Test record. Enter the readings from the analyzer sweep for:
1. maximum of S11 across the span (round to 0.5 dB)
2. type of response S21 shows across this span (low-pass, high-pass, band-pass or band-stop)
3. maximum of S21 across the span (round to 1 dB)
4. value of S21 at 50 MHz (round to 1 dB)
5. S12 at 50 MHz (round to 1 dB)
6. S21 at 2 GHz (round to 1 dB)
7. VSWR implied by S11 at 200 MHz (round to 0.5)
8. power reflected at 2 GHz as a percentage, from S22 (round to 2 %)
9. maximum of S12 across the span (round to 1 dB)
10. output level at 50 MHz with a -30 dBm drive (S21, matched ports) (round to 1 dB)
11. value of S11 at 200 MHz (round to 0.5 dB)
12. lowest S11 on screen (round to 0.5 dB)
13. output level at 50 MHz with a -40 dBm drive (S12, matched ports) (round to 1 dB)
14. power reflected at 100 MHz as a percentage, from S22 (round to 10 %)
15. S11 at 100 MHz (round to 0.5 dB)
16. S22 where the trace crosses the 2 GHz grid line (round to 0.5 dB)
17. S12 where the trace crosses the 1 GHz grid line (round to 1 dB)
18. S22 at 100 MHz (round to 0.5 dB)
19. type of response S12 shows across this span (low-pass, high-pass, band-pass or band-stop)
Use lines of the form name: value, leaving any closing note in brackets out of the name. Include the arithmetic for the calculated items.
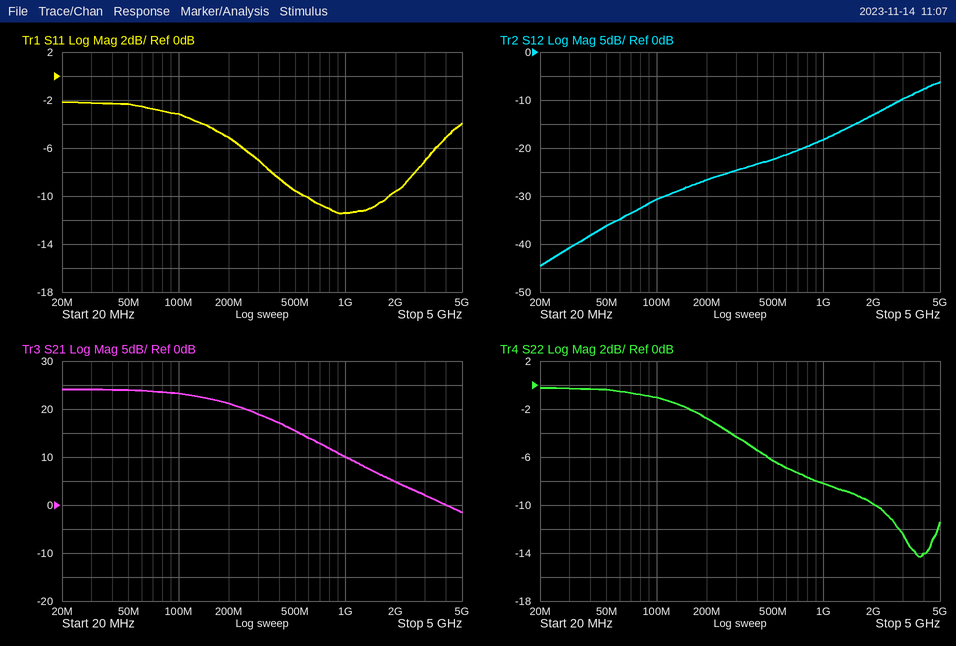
maximum of S11 across the span: -2.0 dB
type of response S21 shows across this span: low-pass
maximum of S21 across the span: 24 dB
value of S21 at 50 MHz: 24 dB
S12 at 50 MHz: -36 dB
S21 at 2 GHz: 5 dB
VSWR implied by S11 at 200 MHz: |Γ| = 10^(-5/20) = 0.5623; VSWR = (1 + 0.5623)/(1 − 0.5623) ≈ 3.57, so 3.5 to the nearest 0.5
power reflected at 2 GHz as a percentage, from S22: 10^(-10/10) ≈ 10 %
maximum of S12 across the span: -6 dB
output level at 50 MHz with a -30 dBm drive (S21, matched ports): -30 dBm + (24 dB) = -6 dBm
value of S11 at 200 MHz: -5.0 dB
lowest S11 on screen: -11.5 dB
output level at 50 MHz with a -40 dBm drive (S12, matched ports): -40 dBm + (-36 dB) = -76 dBm
power reflected at 100 MHz as a percentage, from S22: 10^(-1/10) ≈ 79.4 %, so 80 % to the nearest 10 %
S11 at 100 MHz: -3.0 dB
S22 where the trace crosses the 2 GHz grid line: -10.0 dB
S12 where the trace crosses the 1 GHz grid line: -18 dB
S22 at 100 MHz: -1.0 dB
type of response S12 shows across this span: high-pass
